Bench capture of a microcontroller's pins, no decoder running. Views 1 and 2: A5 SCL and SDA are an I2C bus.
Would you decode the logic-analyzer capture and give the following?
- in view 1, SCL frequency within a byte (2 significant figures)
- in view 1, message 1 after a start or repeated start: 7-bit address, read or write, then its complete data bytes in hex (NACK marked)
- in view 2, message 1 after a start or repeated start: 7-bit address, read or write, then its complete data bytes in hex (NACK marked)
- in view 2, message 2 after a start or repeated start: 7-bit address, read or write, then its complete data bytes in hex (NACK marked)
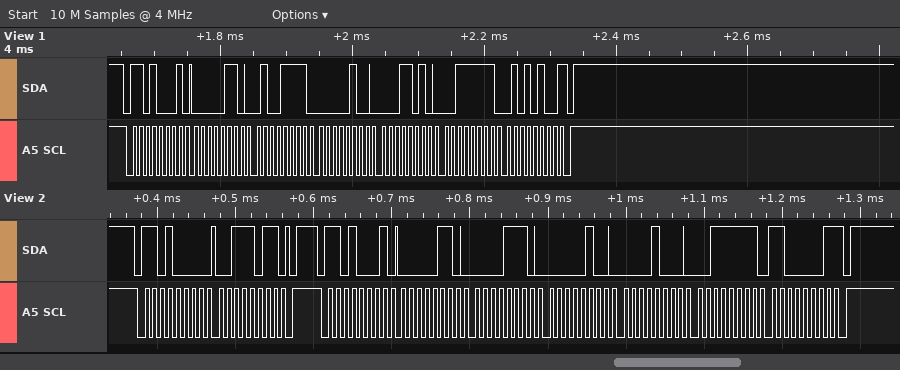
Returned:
100 kHz
0x68 read: 06 4F 04 1A 3F 54 NACK
0x68 write: 3B
0x68 read: 06 0E 04 08 3F C1 NACK
